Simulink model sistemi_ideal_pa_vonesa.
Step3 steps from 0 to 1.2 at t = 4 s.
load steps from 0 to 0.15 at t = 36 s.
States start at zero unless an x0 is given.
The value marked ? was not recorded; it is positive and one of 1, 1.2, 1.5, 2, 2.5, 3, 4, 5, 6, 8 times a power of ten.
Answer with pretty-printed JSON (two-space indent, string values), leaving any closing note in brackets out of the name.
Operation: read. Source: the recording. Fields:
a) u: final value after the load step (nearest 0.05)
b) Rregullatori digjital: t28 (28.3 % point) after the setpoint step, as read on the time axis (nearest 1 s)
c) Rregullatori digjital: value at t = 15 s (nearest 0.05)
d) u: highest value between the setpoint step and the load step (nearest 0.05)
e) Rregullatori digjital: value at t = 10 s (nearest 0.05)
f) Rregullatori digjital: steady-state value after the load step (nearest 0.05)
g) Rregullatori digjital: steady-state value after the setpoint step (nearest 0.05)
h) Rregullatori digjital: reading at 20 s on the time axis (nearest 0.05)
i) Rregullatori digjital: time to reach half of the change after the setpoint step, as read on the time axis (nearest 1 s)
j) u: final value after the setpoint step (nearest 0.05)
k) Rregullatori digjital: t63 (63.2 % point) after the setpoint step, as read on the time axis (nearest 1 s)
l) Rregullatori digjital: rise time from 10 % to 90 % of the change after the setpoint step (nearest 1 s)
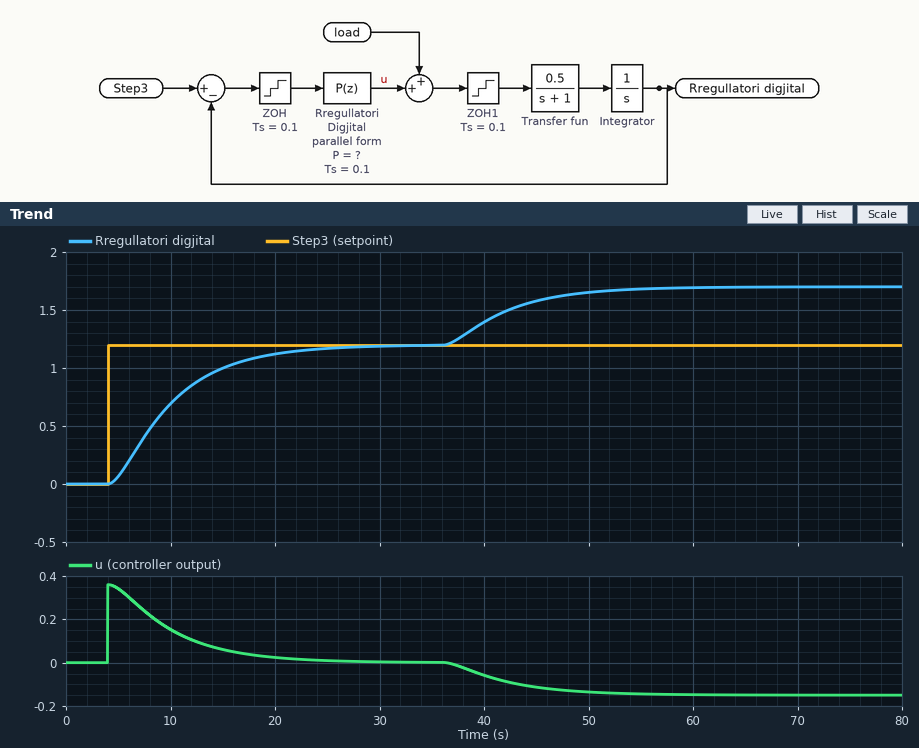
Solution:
{
  "u: final value after the load step": "-0.15",
  "Rregullatori digjital: t28 (28.3 % point) after the setpoint step, as read on the time axis": "7 s",
  "Rregullatori digjital: value at t = 15 s": "1.00",
  "u: highest value between the setpoint step and the load step": "0.35",
  "Rregullatori digjital: value at t = 10 s": "0.70",
  "Rregullatori digjital: steady-state value after the load step": "1.70",
  "Rregullatori digjital: steady-state value after the setpoint step": "1.20",
  "Rregullatori digjital: reading at 20 s on the time axis": "1.10",
  "Rregullatori digjital: time to reach half of the change after the setpoint step, as read on the time axis": "9 s",
  "u: final value after the setpoint step": "0.00",
  "Rregullatori digjital: t63 (63.2 % point) after the setpoint step, as read on the time axis": "11 s",
  "Rregullatori digjital: rise time from 10 % to 90 % of the change after the setpoint step": "12 s"
}
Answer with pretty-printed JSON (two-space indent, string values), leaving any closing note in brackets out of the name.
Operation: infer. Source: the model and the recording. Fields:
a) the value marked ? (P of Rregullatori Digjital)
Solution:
{
  "the value marked ?": "0.3"
}
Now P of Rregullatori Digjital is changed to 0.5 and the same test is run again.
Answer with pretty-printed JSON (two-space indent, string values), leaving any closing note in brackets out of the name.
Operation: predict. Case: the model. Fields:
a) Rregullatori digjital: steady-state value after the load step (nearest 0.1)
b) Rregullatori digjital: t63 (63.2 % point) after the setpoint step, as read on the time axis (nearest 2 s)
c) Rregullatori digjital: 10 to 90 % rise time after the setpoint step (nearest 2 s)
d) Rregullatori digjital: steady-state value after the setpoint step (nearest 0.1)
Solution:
{
  "Rregullatori digjital: steady-state value after the load step": "1.5",
  "Rregullatori digjital: t63 (63.2 % point) after the setpoint step, as read on the time axis": "8 s",
  "Rregullatori digjital: 10 to 90 % rise time after the setpoint step": "6 s",
  "Rregullatori digjital: steady-state value after the setpoint step": "1.2"
}
